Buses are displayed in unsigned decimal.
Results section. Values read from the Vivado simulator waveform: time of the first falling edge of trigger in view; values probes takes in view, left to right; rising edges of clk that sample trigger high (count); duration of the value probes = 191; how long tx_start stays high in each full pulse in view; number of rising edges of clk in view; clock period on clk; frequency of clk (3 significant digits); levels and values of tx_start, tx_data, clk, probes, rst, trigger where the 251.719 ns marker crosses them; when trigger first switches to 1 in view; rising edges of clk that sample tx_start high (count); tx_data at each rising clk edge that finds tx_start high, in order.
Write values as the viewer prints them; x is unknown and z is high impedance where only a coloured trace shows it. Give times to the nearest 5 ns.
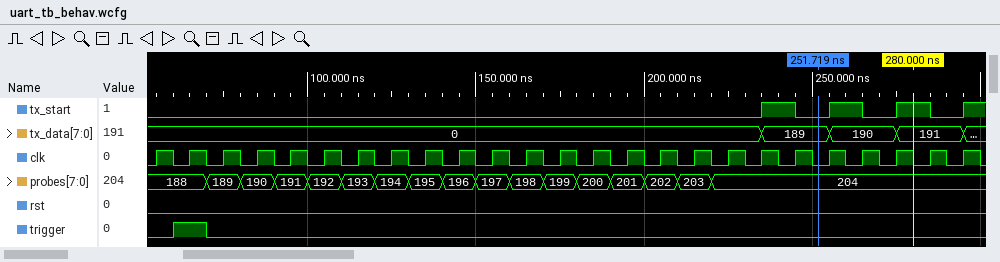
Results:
70 ns
188, 189, 190, 191, 192, 193, 194, 195, 196, 197, 198, 199, 200, 201, 202, 203, 204
1
10 ns
10 ns, 10 ns, 10 ns
25
10 ns
100 MHz
tx_start=0, tx_data=189, clk=0, probes=204, rst=0, trigger=0
60 ns
3
189, 190, 191
